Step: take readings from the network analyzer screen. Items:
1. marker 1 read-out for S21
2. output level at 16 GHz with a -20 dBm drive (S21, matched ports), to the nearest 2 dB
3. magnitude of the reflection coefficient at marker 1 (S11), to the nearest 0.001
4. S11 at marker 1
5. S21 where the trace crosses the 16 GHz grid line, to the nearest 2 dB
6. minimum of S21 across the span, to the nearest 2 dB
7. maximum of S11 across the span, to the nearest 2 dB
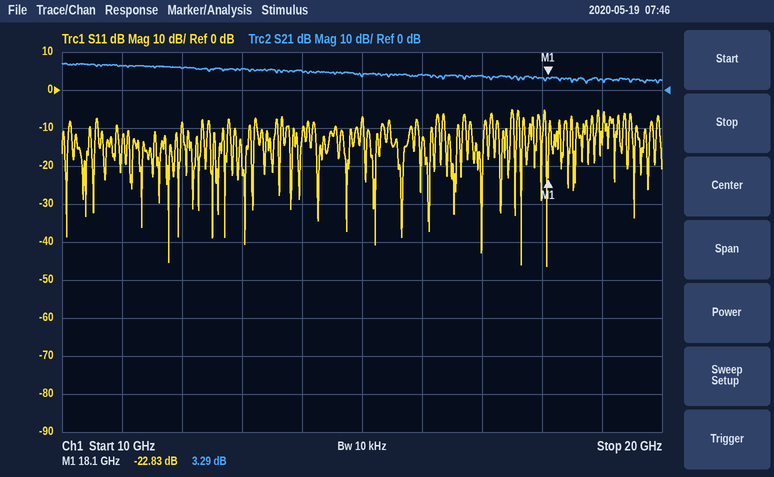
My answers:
3.29 dB
-16 dBm
0.072
-22.83 dB
4 dB
2 dB
-6 dB
